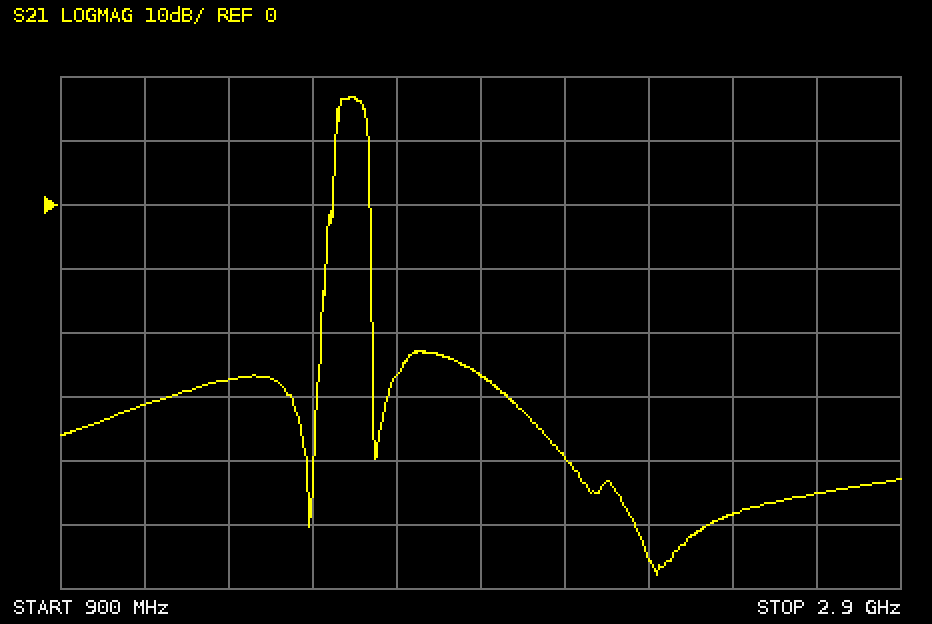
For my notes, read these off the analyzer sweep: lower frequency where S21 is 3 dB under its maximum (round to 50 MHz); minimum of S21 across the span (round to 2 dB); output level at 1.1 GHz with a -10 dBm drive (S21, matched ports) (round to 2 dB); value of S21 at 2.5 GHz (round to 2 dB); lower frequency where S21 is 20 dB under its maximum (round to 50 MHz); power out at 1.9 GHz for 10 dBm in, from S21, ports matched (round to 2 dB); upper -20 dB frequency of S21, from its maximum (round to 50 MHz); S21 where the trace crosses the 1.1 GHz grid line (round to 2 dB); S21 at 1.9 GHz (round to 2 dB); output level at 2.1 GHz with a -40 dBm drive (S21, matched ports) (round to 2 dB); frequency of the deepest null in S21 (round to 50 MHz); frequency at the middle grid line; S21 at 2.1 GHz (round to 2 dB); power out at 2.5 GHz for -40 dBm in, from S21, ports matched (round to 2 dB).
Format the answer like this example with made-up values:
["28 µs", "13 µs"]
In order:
["1.55 GHz", "-58 dB", "-42 dBm", "-48 dB", "1.55 GHz", "-16 dBm", "1.65 GHz", "-32 dB", "-26 dB", "-80 dBm", "2.30 GHz", "1.9 GHz", "-40 dB", "-88 dBm"]
